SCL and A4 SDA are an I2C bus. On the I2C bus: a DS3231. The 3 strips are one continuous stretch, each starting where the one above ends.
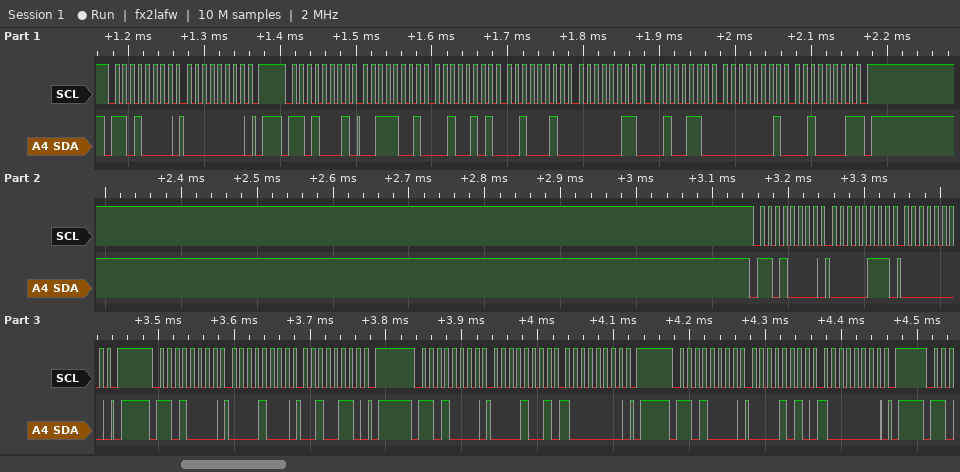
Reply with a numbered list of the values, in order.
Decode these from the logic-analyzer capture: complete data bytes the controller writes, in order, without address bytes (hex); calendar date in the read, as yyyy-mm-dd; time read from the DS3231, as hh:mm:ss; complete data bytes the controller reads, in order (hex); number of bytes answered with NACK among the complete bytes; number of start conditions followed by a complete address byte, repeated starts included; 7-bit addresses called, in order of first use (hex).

1. 00 07 00 08 26 09 80 0A 80
2. 2021-01-26
3. 22:25:39
4. 39 25 22 03 26 01 21
5. 1
6. 6
7. 0x68
